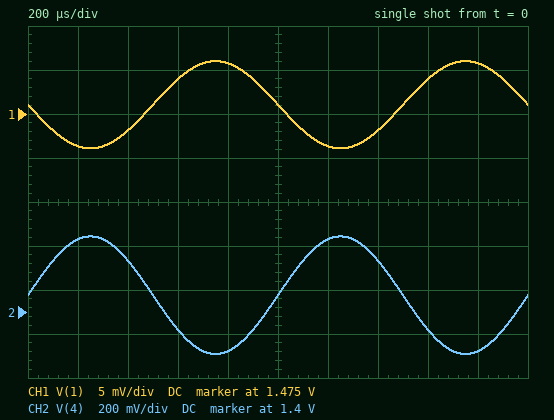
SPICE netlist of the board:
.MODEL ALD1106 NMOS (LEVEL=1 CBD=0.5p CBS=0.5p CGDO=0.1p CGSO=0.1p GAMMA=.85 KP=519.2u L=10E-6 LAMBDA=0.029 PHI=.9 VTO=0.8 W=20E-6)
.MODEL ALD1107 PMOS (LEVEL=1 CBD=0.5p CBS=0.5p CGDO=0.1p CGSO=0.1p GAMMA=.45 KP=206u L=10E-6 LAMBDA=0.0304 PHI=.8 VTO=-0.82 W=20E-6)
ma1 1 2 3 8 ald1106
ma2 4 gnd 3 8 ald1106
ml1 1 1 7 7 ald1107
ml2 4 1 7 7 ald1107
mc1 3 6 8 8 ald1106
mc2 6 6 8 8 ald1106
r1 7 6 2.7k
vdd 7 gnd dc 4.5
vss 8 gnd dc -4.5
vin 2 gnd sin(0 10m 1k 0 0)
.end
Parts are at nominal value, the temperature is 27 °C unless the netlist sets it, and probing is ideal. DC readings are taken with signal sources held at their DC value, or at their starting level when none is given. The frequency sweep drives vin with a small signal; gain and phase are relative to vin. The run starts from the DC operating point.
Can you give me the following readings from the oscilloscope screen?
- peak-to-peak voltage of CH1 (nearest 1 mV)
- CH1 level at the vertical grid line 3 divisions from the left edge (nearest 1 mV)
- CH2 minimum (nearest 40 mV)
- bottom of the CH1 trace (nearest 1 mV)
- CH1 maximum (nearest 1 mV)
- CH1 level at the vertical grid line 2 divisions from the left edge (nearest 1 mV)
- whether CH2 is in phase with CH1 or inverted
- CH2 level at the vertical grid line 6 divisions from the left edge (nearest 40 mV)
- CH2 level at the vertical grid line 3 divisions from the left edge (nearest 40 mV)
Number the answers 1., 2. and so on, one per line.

1. 10 mV
2. 1.479 V
3. 1.20 V
4. 1.471 V
5. 1.481 V
6. 1.473 V
7. inverted
8. 1.72 V
9. 1.32 V
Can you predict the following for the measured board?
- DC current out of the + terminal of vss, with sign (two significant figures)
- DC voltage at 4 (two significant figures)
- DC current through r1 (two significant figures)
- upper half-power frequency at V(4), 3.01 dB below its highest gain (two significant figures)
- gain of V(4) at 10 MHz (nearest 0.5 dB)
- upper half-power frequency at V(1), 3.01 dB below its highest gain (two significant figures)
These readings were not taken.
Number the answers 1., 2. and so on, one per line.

1. -4.5 mA
2. 1.5 V
3. 2.3 mA
4. 23 MHz
5. 28.0 dB
6. 720 MHz
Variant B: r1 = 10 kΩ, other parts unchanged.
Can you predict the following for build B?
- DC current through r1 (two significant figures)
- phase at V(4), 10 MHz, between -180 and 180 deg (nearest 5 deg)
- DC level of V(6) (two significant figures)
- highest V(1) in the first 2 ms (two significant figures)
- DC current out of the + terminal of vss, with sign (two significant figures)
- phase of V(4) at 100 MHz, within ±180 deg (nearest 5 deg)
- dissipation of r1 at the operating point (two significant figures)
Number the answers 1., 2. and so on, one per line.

1. 710 µA
2. -55 deg
3. -2.6 V
4. 2.4 V
5. -1.4 mA
6. -100 deg
7. 5.0 mW
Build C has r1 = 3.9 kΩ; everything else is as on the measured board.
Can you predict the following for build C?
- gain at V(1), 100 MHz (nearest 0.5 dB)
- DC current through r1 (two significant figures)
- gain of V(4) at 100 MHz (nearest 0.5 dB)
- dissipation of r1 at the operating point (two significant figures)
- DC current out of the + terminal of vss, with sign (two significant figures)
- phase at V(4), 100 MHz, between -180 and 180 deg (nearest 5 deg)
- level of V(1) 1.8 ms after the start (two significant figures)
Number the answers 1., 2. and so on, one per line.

1. -2.0 dB
2. 1.7 mA
3. 14.5 dB
4. 11 mW
5. -3.3 mA
6. -90 deg
7. 1.8 V
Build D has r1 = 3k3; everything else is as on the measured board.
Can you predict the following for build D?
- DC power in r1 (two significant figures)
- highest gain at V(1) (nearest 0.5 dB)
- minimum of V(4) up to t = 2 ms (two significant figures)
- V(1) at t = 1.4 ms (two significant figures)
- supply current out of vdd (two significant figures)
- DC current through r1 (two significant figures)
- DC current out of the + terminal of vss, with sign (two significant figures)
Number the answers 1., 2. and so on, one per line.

1. 12 mW
2. -2.0 dB
3. 1.3 V
4. 1.6 V
5. 3.8 mA
6. 1.9 mA
7. -3.8 mA
